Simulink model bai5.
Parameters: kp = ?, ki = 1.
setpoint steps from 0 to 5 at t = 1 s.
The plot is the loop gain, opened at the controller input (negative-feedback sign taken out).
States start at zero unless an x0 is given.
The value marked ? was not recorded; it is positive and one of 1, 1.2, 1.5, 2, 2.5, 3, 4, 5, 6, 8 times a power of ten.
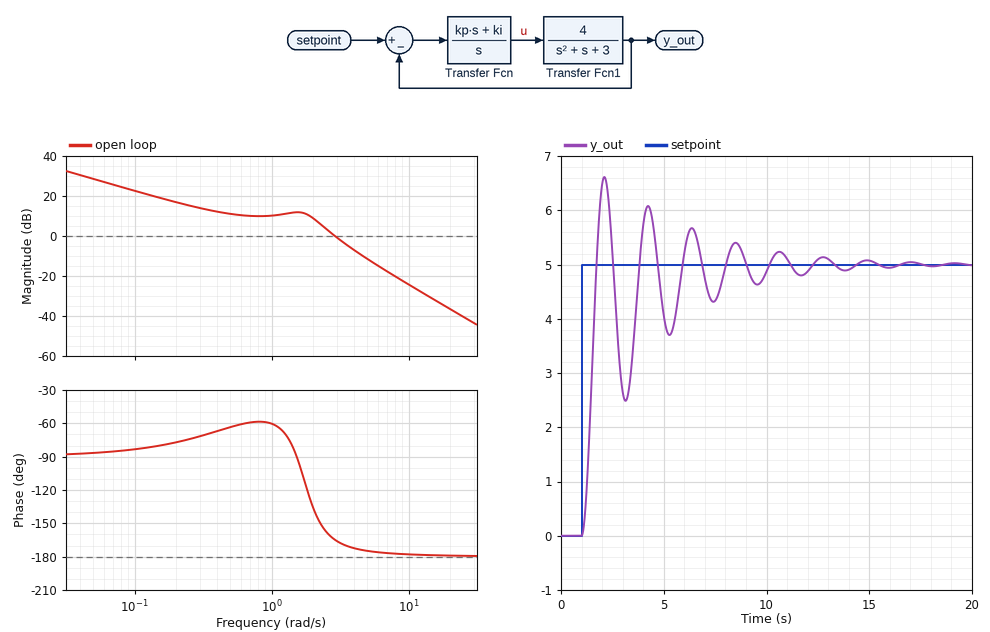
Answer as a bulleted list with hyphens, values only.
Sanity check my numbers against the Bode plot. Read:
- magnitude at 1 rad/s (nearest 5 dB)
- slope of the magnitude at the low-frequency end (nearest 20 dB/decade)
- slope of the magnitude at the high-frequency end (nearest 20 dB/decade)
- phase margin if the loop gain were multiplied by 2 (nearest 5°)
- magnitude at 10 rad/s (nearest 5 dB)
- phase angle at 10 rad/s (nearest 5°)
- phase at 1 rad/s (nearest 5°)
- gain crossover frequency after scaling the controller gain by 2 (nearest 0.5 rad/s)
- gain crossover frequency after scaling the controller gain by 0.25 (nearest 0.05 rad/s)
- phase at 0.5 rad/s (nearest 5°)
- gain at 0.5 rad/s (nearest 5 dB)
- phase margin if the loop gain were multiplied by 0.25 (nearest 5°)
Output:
- 10 dB
- -20 dB/decade
- -40 dB/decade
- 10°
- -25 dB
- -180°
- -60°
- 4.0 rad/s
- 0.40 rad/s
- -65°
- 10 dB
- 115°
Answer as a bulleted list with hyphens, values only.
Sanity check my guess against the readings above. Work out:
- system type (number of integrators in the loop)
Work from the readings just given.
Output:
- 1
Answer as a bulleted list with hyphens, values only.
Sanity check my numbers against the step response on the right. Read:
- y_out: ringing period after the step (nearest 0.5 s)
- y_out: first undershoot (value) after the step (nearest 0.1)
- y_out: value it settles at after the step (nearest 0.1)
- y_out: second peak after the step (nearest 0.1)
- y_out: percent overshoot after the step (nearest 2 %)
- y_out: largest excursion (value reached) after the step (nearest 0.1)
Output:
- 2.0 s
- 2.5
- 5.0
- 6.1
- 32 %
- 6.6
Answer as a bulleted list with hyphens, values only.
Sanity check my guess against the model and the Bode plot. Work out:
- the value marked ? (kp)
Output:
- 1.5
